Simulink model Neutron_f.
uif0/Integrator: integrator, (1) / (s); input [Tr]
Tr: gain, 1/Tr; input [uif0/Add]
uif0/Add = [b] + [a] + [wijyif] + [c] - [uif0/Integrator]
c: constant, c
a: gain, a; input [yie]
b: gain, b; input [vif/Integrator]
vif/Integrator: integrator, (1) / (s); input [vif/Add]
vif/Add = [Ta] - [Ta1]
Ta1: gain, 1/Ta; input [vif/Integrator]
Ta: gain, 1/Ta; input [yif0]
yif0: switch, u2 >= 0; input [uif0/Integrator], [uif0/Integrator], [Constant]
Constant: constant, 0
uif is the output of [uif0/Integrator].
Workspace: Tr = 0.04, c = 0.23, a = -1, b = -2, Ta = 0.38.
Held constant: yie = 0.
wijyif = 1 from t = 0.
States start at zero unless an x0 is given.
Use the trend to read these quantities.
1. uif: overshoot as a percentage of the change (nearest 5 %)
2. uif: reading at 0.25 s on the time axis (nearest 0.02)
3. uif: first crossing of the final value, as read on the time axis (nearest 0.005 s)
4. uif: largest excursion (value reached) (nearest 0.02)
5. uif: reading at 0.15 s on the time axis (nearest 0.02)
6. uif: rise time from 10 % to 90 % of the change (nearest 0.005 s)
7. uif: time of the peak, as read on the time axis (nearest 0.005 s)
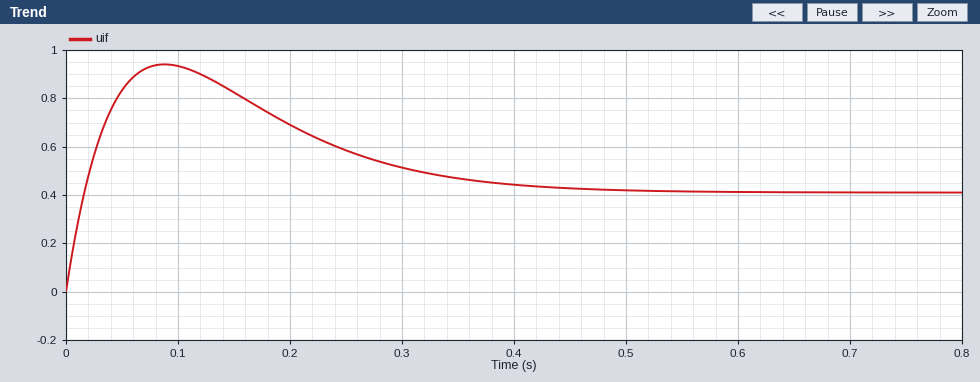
130 %
0.58
0.015 s
0.94
0.82
0.015 s
0.090 s
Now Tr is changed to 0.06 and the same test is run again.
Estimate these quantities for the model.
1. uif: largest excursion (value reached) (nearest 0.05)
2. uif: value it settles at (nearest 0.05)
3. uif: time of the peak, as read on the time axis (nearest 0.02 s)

0.90
0.40
0.12 s
